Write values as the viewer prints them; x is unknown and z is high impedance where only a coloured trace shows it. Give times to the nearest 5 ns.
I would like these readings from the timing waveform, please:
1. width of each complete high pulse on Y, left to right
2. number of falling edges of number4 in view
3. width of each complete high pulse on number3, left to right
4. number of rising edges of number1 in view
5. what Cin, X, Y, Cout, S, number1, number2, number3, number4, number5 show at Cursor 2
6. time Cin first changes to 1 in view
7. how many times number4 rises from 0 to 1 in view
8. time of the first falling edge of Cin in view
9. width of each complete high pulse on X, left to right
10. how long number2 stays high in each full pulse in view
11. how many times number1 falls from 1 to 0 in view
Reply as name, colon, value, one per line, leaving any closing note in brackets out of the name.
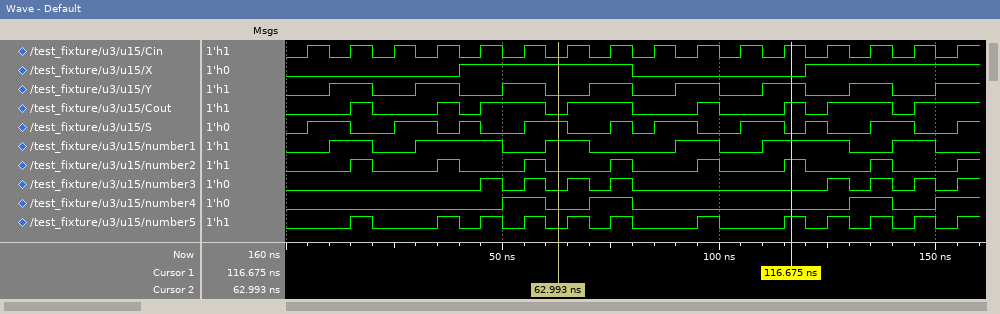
width of each complete high pulse on Y, left to right: 10 ns, 10 ns, 10 ns, 10 ns, 10 ns, 10 ns, 10 ns
number of falling edges of number4 in view: 3
width of each complete high pulse on number3, left to right: 5 ns, 5 ns, 5 ns, 5 ns, 5 ns, 5 ns, 5 ns
number of rising edges of number1 in view: 6
what Cin, X, Y, Cout, S, number1, number2, number3, number4, number5 show at Cursor 2: Cin=0, X=1, Y=0, Cout=0, S=1, number1=1, number2=0, number3=0, number4=0, number5=0
time Cin first changes to 1 in view: 5 ns
how many times number4 rises from 0 to 1 in view: 4
time of the first falling edge of Cin in view: 10 ns
width of each complete high pulse on X, left to right: 40 ns
how long number2 stays high in each full pulse in view: 5 ns, 5 ns, 5 ns, 5 ns, 5 ns, 5 ns, 5 ns
how many times number1 falls from 1 to 0 in view: 6
